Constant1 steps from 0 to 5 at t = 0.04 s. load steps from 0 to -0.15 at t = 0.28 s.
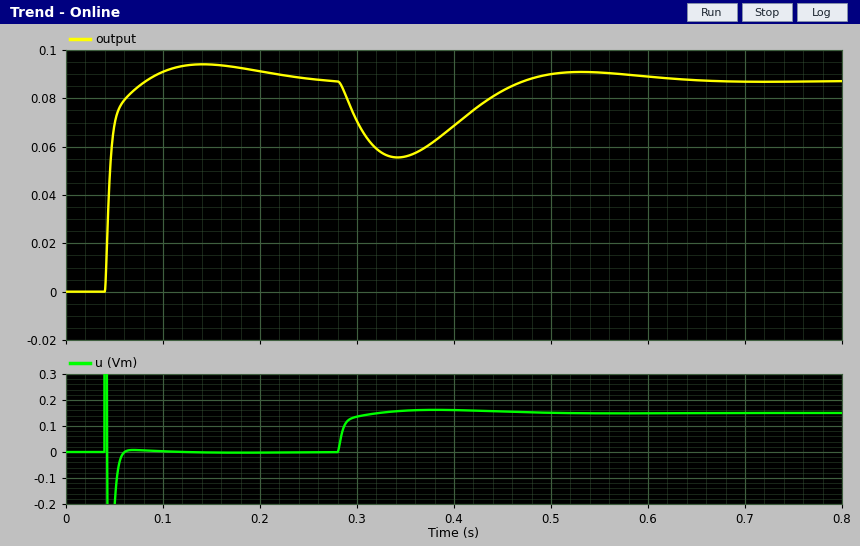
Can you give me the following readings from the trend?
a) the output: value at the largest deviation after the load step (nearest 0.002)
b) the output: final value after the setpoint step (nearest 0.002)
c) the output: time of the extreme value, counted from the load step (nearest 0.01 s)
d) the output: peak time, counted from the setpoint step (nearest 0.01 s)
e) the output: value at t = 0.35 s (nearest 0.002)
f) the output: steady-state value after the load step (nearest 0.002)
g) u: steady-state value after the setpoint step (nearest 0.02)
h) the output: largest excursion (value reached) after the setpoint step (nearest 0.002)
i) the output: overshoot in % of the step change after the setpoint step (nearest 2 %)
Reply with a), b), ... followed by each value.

a) 0.056
b) 0.088
c) 0.06 s
d) 0.10 s
e) 0.056
f) 0.088
g) 0.00
h) 0.094
i) 8 %
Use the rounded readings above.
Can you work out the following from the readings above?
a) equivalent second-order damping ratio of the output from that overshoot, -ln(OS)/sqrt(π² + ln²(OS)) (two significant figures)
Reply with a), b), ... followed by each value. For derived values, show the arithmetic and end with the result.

a) ln(0.08) = -2.526; 2.526 / sqrt(9.870 + 6.379) = 0.63
